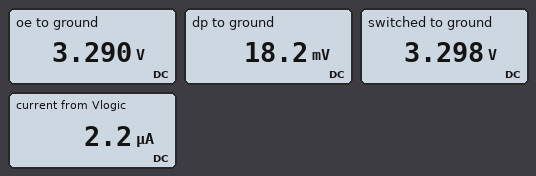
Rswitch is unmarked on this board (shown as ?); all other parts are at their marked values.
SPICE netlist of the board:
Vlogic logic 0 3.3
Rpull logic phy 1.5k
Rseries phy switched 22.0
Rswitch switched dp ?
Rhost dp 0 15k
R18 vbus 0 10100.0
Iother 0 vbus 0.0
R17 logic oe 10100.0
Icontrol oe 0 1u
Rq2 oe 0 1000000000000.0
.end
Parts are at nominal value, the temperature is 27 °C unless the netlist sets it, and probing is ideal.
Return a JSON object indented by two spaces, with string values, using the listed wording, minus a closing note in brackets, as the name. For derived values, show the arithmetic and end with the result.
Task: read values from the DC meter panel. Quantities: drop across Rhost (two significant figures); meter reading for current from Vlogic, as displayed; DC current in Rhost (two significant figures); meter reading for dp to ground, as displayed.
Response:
{
  "drop across Rhost": "18.2 mV = 18 mV",
  "meter reading for current from Vlogic, as displayed": "2.2 µA",
  "DC current in Rhost": "(18.2 mV) / 15 kΩ = 1.2 µA",
  "meter reading for dp to ground, as displayed": "18.2 mV"
}
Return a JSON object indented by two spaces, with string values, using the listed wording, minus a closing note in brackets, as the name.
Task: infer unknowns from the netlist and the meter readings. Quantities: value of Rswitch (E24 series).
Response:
{
  "value of Rswitch": "2.7 MΩ"
}
